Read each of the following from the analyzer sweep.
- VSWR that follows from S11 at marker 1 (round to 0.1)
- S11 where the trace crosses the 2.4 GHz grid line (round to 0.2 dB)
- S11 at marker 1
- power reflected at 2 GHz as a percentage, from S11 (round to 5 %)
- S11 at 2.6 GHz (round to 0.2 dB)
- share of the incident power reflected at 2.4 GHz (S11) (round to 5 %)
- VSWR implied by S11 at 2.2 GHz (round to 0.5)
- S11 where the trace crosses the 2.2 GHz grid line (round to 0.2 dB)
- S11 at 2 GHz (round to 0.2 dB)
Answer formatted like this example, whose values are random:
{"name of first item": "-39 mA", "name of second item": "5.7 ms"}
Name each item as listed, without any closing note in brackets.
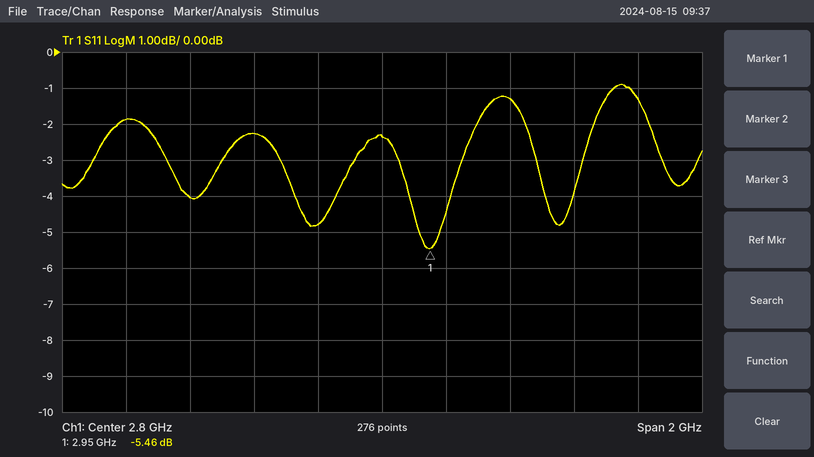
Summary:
{"VSWR that follows from S11 at marker 1": "3.3", "S11 where the trace crosses the 2.4 GHz grid line": "-2.2 dB", "S11 at marker 1": "-5.46 dB", "power reflected at 2 GHz as a percentage, from S11": "65 %", "S11 at 2.6 GHz": "-4.8 dB", "share of the incident power reflected at 2.4 GHz (S11)": "60 %", "VSWR implied by S11 at 2.2 GHz": "4.5", "S11 where the trace crosses the 2.2 GHz grid line": "-4.0 dB", "S11 at 2 GHz": "-1.8 dB"}
